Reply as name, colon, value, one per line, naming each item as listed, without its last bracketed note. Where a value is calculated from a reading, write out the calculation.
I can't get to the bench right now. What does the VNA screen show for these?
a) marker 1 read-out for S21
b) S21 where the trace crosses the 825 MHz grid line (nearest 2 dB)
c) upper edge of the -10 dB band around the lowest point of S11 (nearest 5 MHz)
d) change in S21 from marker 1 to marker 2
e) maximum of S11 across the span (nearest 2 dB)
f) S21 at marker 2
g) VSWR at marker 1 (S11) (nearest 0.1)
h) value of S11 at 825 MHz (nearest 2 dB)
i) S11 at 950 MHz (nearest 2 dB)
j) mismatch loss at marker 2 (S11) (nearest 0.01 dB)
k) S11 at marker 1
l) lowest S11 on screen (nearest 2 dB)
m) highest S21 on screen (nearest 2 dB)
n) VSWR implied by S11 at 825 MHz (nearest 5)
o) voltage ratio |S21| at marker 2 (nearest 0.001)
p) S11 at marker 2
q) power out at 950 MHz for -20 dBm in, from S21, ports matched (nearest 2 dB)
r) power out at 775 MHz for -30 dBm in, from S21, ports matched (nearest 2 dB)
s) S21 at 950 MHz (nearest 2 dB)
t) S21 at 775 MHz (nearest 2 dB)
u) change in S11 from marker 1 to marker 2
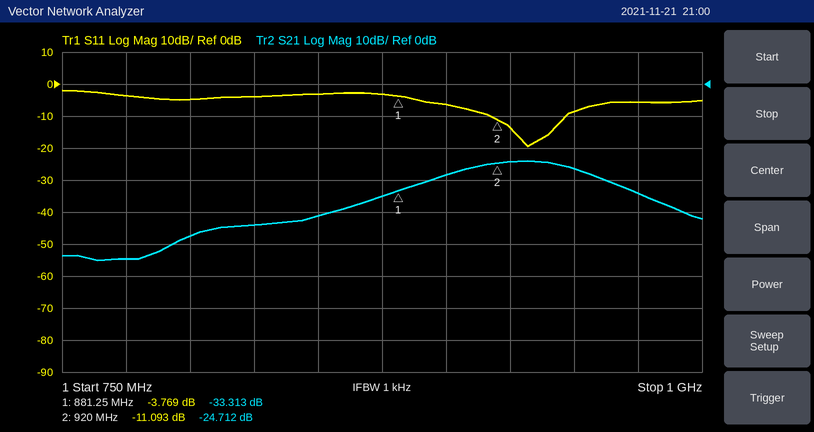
marker 1 read-out for S21: -33.313 dB
S21 where the trace crosses the 825 MHz grid line: -44 dB
upper edge of the -10 dB band around the lowest point of S11: 945 MHz
change in S21 from marker 1 to marker 2: -24.712 − (-33.313) = 8.601 dB
maximum of S11 across the span: -2 dB
S21 at marker 2: -24.712 dB
VSWR at marker 1 (S11): (1 + 0.6480)/(1 − 0.6480) ≈ 4.7
value of S11 at 825 MHz: -4 dB
S11 at 950 MHz: -8 dB
mismatch loss at marker 2 (S11): −10 log10(1 − 10^(-11.093/10)) ≈ 0.35 dB
S11 at marker 1: -3.769 dB
lowest S11 on screen: -20 dB
highest S21 on screen: -24 dB
VSWR implied by S11 at 825 MHz: |Γ| = 10^(-4/20) = 0.6310; VSWR = (1 + 0.6310)/(1 − 0.6310) ≈ 4.42, so 5 to the nearest 5
voltage ratio |S21| at marker 2: 10^(-24.712/20) ≈ 0.058
S11 at marker 2: -11.093 dB
power out at 950 MHz for -20 dBm in, from S21, ports matched: -20 dBm + (-26 dB) = -46 dBm
power out at 775 MHz for -30 dBm in, from S21, ports matched: -30 dBm + (-54 dB) = -84 dBm
S21 at 950 MHz: -26 dB
S21 at 775 MHz: -54 dB
change in S11 from marker 1 to marker 2: -11.093 − (-3.769) = -7.324 dB
